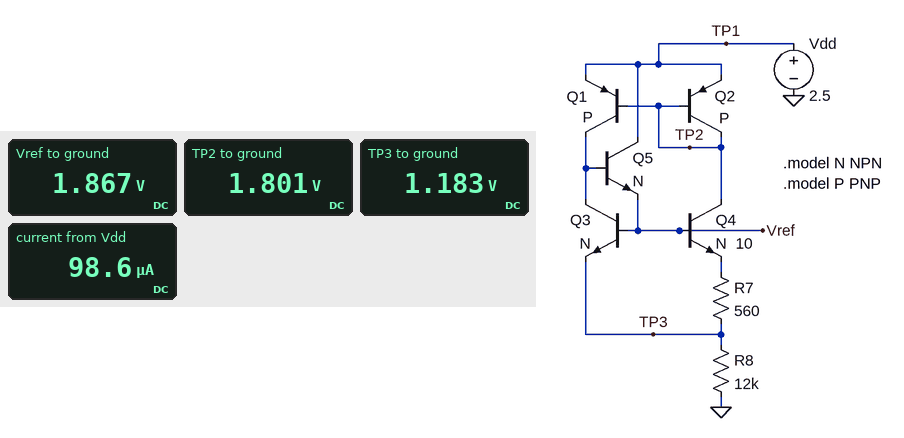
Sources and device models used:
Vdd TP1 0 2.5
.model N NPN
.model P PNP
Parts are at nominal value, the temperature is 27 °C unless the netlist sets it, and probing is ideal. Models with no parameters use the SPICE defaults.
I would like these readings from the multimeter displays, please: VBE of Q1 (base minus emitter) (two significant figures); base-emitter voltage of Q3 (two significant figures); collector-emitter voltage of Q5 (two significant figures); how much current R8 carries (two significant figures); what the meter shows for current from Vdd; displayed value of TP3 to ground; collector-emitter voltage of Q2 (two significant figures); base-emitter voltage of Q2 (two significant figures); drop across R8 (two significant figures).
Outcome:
-700 mV
680 mV
630 mV
99 µA
98.6 µA
1.183 V
-700 mV
-700 mV
1.2 V
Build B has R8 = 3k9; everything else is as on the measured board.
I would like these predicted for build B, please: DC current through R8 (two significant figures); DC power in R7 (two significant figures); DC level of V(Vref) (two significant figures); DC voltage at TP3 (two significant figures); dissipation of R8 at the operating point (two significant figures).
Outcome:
210 µA
6.2 µW
1.5 V
810 mV
170 µW
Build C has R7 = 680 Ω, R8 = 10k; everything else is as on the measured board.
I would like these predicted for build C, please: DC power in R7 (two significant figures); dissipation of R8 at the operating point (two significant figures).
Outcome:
3.4 µW
130 µW
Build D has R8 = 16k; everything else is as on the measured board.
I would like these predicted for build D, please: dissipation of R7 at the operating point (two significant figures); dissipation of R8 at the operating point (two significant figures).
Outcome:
1.8 µW
91 µW
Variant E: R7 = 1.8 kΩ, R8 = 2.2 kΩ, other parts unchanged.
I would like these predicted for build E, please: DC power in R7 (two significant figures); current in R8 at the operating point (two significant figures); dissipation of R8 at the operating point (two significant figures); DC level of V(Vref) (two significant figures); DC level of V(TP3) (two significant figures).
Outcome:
1.9 µW
65 µA
9.3 µW
830 mV
140 mV
